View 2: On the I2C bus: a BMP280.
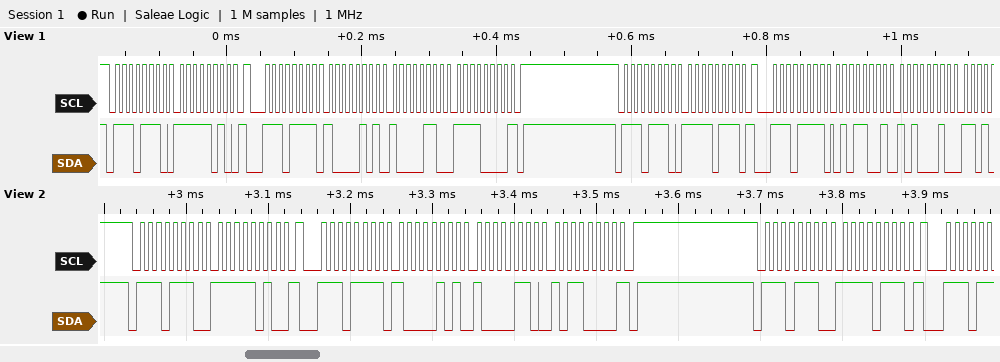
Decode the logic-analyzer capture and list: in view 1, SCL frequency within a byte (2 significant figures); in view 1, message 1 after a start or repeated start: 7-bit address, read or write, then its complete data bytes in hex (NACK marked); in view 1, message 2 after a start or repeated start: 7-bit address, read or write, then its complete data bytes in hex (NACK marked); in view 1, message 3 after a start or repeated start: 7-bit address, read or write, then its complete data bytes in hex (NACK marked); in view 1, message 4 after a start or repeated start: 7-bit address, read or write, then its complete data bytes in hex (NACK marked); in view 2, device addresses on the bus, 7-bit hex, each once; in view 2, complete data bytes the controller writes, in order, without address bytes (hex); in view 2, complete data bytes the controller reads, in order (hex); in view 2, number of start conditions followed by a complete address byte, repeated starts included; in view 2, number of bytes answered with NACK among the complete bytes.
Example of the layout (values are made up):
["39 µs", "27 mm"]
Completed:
["100 kHz", "0x77 write: FA", "0x77 read: 85 86 F0 NACK", "0x77 write: F7", "0x77 read: 59 A2", "0x77", "FA F7", "85 86 B0", "3", "1"]
